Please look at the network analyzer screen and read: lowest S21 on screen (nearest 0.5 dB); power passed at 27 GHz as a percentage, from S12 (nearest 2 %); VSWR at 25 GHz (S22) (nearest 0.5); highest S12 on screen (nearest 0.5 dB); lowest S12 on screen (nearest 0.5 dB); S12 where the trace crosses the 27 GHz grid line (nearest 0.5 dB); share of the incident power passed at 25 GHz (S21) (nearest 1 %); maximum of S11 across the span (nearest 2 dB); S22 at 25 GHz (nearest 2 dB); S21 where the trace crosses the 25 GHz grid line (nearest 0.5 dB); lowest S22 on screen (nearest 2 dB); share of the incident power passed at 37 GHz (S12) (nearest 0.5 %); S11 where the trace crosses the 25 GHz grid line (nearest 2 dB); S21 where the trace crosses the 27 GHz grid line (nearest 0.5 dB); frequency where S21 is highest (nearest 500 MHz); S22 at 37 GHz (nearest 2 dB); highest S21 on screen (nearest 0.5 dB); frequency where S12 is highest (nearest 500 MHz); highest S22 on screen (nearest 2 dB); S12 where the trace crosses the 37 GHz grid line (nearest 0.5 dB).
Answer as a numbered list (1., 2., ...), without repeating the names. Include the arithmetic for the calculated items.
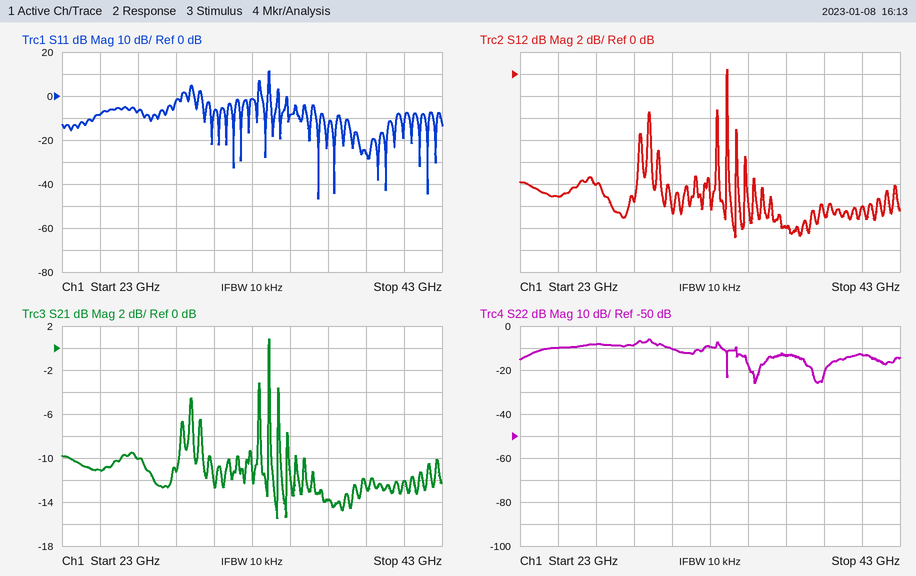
1. -15.5 dB
2. 10^(-10/10) ≈ 10 %
3. |Γ| = 10^(-10/20) = 0.3162; VSWR = (1 + 0.3162)/(1 − 0.3162) ≈ 1.92, so 2.0 to the nearest 0.5
4. 0.5 dB
5. -15.0 dB
6. -10.0 dB
7. 10^(-11/10) ≈ 8 %
8. 12 dB
9. -10 dB
10. -11.0 dB
11. -26 dB
12. 10^(-14/10) ≈ 4.0 %
13. -8 dB
14. -10.0 dB
15. 34.0 GHz
16. -14 dB
17. 1.0 dB
18. 34.0 GHz
19. -6 dB
20. -14.0 dB
